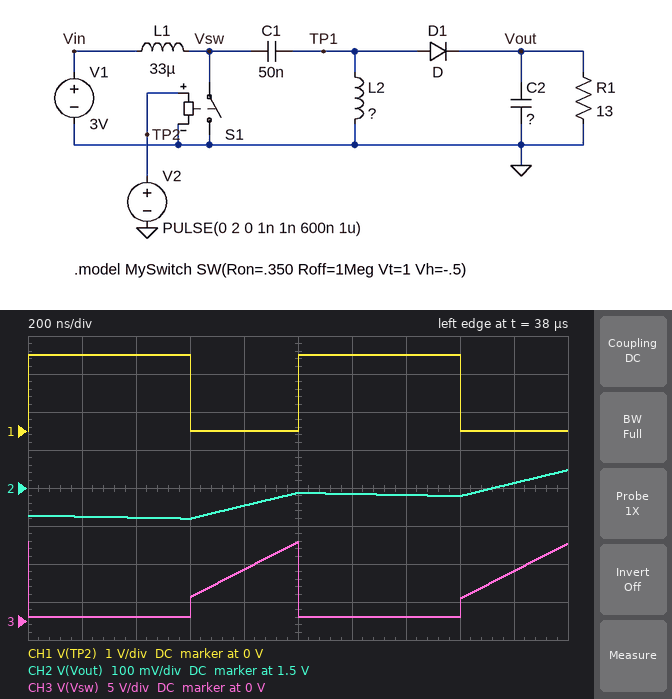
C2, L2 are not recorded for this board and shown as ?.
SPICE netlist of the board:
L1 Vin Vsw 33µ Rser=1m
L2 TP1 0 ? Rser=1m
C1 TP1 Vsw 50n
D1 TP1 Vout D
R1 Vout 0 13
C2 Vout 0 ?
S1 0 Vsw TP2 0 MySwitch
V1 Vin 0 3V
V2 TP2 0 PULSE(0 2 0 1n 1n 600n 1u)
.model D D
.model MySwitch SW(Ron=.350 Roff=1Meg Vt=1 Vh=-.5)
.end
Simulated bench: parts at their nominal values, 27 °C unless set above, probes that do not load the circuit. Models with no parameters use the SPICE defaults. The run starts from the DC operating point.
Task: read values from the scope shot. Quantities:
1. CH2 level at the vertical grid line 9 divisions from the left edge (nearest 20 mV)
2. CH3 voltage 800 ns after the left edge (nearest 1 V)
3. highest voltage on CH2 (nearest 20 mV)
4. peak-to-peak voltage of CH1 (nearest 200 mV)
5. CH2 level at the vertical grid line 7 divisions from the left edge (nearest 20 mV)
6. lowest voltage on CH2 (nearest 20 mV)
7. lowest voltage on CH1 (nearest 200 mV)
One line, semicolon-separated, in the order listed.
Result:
1.52 V; 7 V; 1.54 V; 2.0 V; 1.48 V; 1.42 V; 0 V
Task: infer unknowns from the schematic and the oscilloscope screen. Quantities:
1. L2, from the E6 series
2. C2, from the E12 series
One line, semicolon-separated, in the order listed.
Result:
100 µH; 8.2 µF
